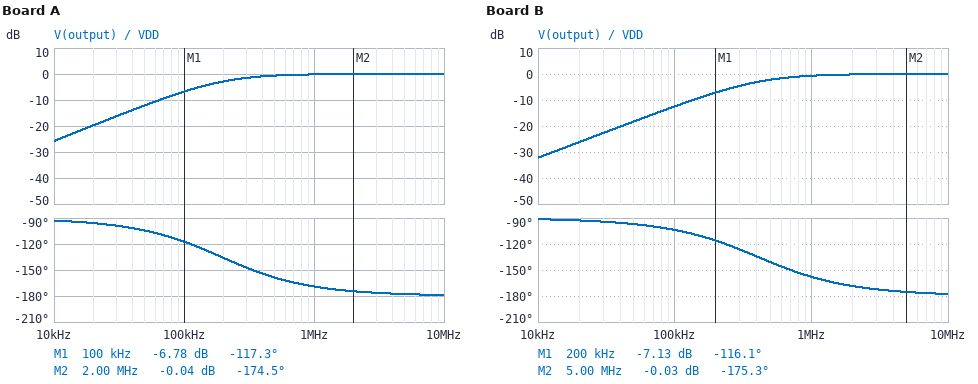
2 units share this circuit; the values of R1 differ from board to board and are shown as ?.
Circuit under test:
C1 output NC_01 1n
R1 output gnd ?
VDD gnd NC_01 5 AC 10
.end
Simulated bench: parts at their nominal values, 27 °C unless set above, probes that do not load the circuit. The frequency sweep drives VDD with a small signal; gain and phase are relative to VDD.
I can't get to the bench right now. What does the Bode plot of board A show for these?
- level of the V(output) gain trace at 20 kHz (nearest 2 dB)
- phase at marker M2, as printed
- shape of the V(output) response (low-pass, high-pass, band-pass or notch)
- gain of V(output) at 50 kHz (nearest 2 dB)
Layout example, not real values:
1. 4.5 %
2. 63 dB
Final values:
1. -20 dB
2. -174.5 deg
3. high-pass
4. -12 dB
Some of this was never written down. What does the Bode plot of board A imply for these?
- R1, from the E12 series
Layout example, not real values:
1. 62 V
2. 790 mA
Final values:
1. 820 Ω
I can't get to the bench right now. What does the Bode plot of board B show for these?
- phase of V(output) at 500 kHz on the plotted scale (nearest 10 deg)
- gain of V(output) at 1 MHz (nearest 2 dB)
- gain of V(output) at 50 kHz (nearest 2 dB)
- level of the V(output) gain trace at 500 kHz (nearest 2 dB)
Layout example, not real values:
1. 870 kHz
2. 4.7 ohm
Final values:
1. -140 deg
2. 0 dB
3. -18 dB
4. -2 dB
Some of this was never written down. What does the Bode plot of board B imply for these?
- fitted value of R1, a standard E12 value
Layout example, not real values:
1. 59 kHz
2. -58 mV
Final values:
1. 390 Ω
